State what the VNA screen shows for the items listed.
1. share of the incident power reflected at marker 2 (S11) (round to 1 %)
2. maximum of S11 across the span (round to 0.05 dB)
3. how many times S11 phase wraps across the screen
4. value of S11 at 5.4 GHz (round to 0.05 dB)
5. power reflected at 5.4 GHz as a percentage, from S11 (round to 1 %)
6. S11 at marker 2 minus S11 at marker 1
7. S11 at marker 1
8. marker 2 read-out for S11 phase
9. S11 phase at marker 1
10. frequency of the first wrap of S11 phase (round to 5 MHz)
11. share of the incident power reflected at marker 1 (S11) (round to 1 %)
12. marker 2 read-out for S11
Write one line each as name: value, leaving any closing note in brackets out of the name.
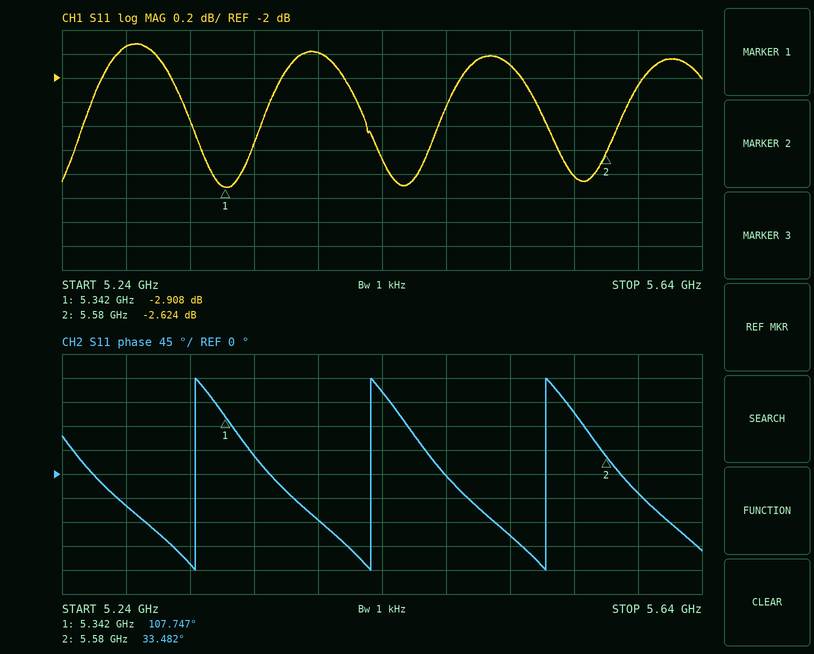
share of the incident power reflected at marker 2 (S11): 55 %
maximum of S11 across the span: -1.70 dB
how many times S11 phase wraps across the screen: 3
value of S11 at 5.4 GHz: -1.80 dB
power reflected at 5.4 GHz as a percentage, from S11: 66 %
S11 at marker 2 minus S11 at marker 1: 0.284 dB
S11 at marker 1: -2.908 dB
marker 2 read-out for S11 phase: 33.482°
S11 phase at marker 1: 107.747°
frequency of the first wrap of S11 phase: 5.325 GHz
share of the incident power reflected at marker 1 (S11): 51 %
marker 2 read-out for S11: -2.624 dB
